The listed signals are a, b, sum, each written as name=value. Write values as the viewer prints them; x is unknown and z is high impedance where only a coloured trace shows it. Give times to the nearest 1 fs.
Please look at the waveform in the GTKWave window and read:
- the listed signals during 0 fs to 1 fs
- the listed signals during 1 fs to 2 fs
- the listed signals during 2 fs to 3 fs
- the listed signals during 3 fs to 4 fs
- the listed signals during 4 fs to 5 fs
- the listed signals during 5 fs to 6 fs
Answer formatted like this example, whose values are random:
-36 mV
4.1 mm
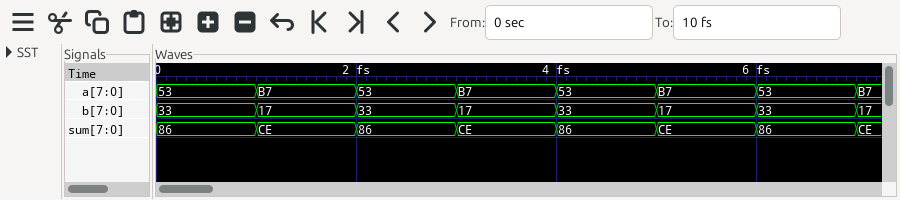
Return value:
a=53, b=33, sum=86
a=B7, b=17, sum=CE
a=53, b=33, sum=86
a=B7, b=17, sum=CE
a=53, b=33, sum=86
a=B7, b=17, sum=CE
